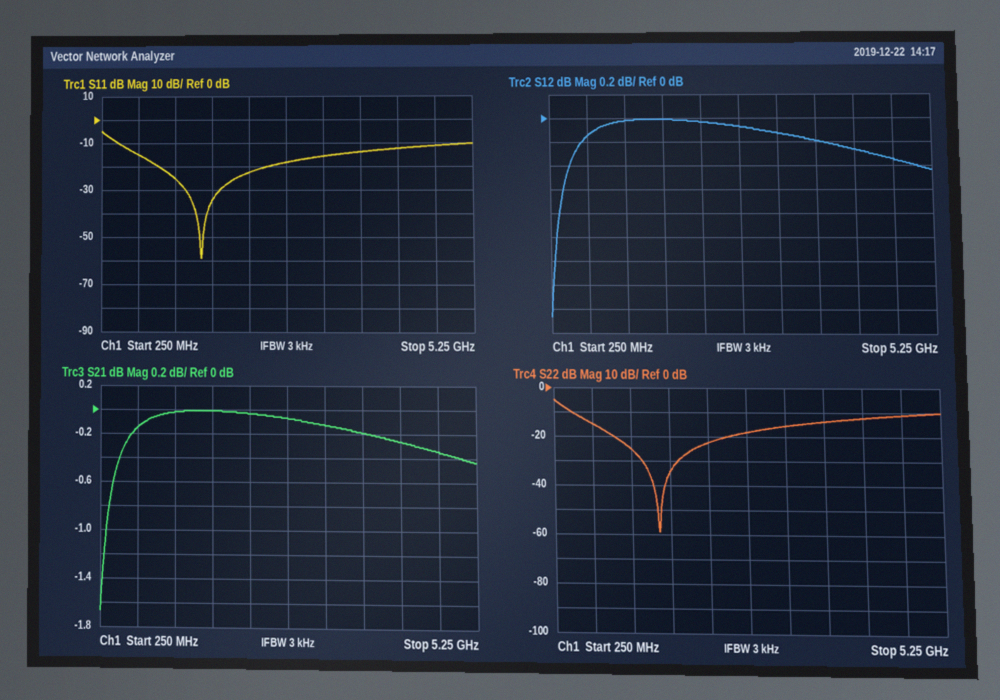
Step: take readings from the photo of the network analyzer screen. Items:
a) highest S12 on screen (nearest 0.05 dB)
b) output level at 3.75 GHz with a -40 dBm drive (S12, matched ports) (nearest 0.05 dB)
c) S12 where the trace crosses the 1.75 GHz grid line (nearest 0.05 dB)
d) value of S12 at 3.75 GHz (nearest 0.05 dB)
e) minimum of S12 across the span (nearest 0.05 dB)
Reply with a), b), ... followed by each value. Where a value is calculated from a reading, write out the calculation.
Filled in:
a) 0.00 dB
b) -40 dBm + (-0.20 dB) = -40.20 dBm
c) 0.00 dB
d) -0.20 dB
e) -1.65 dB
